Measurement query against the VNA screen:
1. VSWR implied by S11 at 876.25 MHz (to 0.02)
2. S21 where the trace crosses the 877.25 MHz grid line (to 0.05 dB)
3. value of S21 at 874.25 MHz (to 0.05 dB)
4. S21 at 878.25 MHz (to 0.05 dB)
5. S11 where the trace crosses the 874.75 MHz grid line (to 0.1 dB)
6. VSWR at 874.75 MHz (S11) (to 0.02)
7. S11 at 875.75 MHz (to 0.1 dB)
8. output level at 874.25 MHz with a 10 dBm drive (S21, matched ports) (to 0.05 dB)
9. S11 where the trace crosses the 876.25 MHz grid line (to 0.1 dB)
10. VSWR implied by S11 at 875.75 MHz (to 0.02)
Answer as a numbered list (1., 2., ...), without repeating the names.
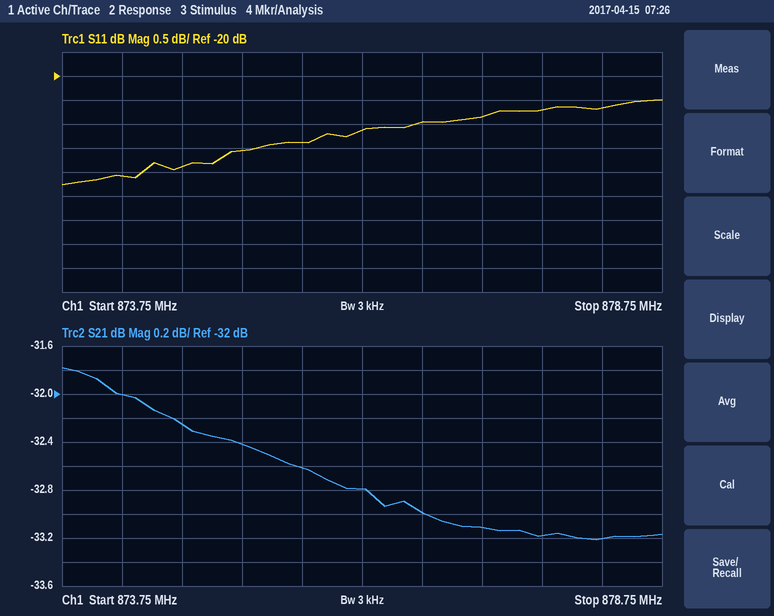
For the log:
1. 1.20
2. -33.10 dB
3. -32.00 dB
4. -33.20 dB
5. -21.9 dB
6. 1.18
7. -21.4 dB
8. -22.00 dBm
9. -21.1 dB
10. 1.18
